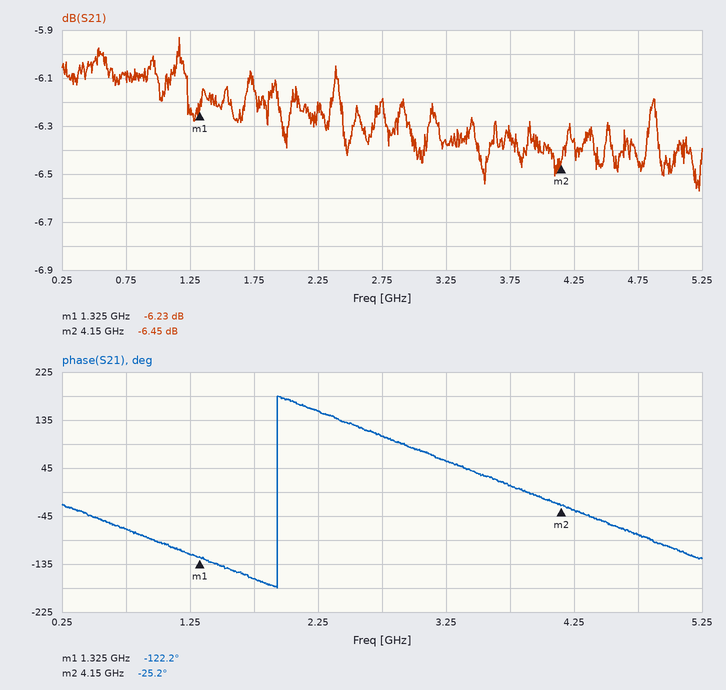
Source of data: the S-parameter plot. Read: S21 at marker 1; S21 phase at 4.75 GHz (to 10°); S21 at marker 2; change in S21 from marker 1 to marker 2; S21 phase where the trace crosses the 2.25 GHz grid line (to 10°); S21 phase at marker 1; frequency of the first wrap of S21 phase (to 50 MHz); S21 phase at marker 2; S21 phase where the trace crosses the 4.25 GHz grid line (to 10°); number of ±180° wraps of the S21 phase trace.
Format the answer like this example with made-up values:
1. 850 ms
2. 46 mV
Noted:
1. -6.23 dB
2. -80°
3. -6.45 dB
4. -0.22 dB
5. 150°
6. -122.2°
7. 1.95 GHz
8. -25.2°
9. -30°
10. 1
